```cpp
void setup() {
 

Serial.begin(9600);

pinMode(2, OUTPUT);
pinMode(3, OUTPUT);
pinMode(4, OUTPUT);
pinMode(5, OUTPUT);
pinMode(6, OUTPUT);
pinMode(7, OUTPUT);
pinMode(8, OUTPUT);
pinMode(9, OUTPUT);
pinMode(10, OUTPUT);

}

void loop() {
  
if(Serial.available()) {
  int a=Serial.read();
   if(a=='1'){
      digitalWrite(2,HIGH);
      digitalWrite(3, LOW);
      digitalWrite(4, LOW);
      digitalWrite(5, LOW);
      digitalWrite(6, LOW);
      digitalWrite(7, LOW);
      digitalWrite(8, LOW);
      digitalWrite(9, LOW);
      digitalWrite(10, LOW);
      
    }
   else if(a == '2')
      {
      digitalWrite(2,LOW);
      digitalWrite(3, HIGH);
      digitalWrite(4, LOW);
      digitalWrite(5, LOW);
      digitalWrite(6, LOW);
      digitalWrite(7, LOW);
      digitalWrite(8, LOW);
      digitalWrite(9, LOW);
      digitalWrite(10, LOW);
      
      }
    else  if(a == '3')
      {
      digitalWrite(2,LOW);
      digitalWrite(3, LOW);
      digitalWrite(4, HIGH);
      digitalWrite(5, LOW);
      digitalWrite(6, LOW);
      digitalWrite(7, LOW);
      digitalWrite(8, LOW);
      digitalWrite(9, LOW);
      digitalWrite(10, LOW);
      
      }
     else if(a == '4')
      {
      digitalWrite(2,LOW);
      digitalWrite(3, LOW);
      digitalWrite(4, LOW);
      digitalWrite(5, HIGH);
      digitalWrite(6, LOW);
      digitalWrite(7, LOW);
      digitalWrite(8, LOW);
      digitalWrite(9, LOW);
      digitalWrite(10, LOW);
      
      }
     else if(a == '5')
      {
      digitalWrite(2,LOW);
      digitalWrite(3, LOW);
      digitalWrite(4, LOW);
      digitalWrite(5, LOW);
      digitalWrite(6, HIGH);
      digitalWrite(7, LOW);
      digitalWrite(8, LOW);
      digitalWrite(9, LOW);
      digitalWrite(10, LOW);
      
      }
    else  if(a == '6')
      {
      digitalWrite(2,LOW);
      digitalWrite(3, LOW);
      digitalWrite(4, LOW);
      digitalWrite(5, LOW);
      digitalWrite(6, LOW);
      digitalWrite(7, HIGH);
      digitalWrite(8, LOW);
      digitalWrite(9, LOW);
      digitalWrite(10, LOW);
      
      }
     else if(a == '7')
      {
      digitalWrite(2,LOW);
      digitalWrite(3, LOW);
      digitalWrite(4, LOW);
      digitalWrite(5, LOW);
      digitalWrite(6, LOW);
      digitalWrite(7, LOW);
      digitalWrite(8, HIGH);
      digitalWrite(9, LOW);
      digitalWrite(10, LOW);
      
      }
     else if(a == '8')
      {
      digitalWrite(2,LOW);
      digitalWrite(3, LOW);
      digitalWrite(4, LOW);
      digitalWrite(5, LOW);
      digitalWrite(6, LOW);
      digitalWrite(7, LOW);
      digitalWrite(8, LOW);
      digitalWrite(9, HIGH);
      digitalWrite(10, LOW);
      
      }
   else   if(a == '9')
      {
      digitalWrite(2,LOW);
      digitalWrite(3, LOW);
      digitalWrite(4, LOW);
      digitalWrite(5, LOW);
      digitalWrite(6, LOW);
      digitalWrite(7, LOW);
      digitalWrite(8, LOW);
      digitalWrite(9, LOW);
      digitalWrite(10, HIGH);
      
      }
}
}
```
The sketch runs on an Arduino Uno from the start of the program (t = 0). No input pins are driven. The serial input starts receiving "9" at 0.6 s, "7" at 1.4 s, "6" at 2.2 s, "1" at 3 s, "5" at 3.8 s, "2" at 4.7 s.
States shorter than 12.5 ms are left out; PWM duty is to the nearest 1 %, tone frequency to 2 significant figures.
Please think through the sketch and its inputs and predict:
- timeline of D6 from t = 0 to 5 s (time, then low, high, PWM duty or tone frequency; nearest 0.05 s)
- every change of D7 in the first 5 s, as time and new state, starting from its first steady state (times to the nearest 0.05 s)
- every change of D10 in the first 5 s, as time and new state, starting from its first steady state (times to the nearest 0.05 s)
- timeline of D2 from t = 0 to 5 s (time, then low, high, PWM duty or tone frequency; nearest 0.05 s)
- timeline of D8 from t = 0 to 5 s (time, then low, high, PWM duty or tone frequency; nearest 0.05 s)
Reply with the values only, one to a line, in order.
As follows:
0 s low; 3.8 s high; 4.7 s low
0 s low; 2.2 s high; 3 s low
0 s low; 0.6 s high; 1.4 s low
0 s low; 3 s high; 3.8 s low
0 s low; 1.4 s high; 2.2 s low
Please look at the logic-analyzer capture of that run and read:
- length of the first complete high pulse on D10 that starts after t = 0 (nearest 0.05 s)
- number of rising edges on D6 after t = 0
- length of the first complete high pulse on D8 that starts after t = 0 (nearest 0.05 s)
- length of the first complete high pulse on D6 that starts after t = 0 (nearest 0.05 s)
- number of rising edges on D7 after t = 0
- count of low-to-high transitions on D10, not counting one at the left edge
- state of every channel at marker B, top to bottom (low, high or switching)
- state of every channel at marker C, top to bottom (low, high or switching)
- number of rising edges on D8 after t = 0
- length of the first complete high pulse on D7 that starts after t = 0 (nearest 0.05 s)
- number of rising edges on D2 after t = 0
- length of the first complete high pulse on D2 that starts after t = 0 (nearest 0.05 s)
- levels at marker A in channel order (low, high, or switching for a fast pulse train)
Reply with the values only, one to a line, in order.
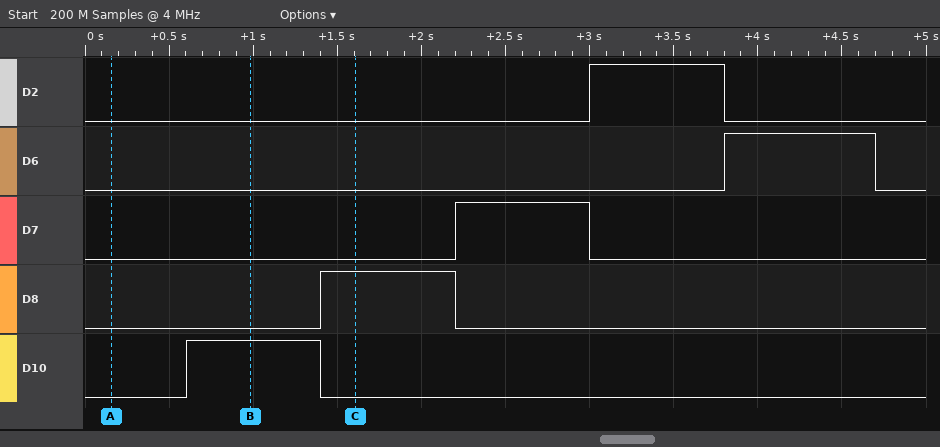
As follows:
0.80 s
1
0.80 s
0.90 s
1
1
D2 low, D6 low, D7 low, D8 low, D10 high
D2 low, D6 low, D7 low, D8 high, D10 low
1
0.80 s
1
0.80 s
D2 low, D6 low, D7 low, D8 low, D10 low
